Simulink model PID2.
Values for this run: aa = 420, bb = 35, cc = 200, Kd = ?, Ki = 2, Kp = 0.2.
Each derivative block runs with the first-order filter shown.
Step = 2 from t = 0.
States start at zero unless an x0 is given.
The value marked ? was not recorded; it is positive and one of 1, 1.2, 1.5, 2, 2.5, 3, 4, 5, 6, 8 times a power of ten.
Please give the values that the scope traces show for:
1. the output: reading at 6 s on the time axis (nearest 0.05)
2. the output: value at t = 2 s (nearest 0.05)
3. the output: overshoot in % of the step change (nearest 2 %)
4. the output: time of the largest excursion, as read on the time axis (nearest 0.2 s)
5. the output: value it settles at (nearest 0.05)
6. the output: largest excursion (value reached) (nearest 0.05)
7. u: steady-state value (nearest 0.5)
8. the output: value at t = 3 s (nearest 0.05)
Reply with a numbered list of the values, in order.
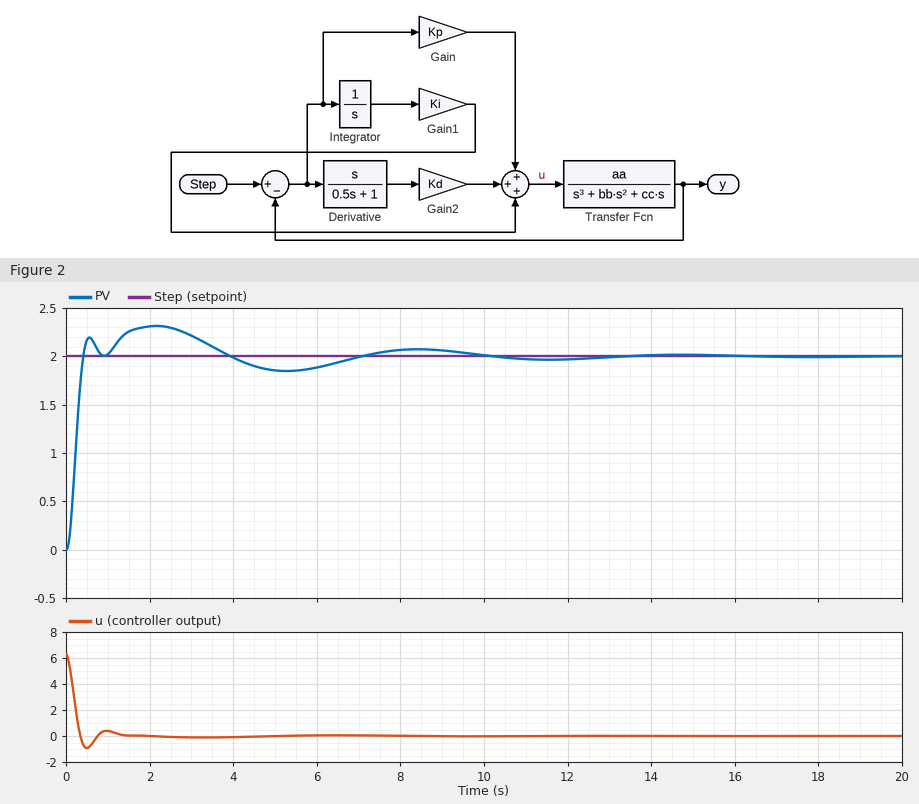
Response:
1. 1.90
2. 2.30
3. 16 %
4. 2.2 s
5. 2.00
6. 2.30
7. 0.0
8. 2.20
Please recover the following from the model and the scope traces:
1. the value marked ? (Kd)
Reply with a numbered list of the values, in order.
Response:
1. 1.5
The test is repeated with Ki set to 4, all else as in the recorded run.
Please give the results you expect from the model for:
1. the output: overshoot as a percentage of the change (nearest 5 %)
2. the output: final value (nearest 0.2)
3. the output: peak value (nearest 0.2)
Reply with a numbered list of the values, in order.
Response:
1. 25 %
2. 2.0
3. 2.6
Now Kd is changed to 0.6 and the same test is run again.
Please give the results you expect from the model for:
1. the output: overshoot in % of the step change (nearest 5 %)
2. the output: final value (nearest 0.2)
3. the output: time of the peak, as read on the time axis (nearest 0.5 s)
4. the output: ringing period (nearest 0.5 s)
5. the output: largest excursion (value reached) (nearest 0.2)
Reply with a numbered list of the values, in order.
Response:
1. 40 %
2. 2.0
3. 1.5 s
4. 4.5 s
5. 2.8
